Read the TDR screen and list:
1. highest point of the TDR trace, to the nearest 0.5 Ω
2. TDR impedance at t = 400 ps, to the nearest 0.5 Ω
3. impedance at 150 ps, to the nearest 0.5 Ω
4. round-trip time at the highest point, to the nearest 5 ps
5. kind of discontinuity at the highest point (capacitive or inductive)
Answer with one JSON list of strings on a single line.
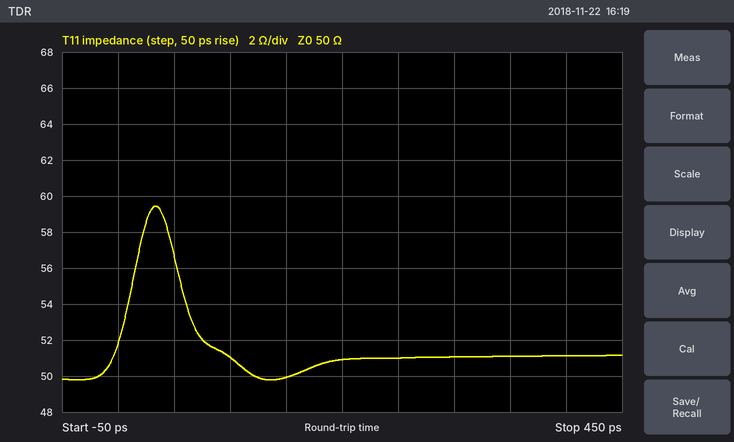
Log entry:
["59.5 Ω", "51.0 Ω", "50.0 Ω", "35 ps", "inductive"]
